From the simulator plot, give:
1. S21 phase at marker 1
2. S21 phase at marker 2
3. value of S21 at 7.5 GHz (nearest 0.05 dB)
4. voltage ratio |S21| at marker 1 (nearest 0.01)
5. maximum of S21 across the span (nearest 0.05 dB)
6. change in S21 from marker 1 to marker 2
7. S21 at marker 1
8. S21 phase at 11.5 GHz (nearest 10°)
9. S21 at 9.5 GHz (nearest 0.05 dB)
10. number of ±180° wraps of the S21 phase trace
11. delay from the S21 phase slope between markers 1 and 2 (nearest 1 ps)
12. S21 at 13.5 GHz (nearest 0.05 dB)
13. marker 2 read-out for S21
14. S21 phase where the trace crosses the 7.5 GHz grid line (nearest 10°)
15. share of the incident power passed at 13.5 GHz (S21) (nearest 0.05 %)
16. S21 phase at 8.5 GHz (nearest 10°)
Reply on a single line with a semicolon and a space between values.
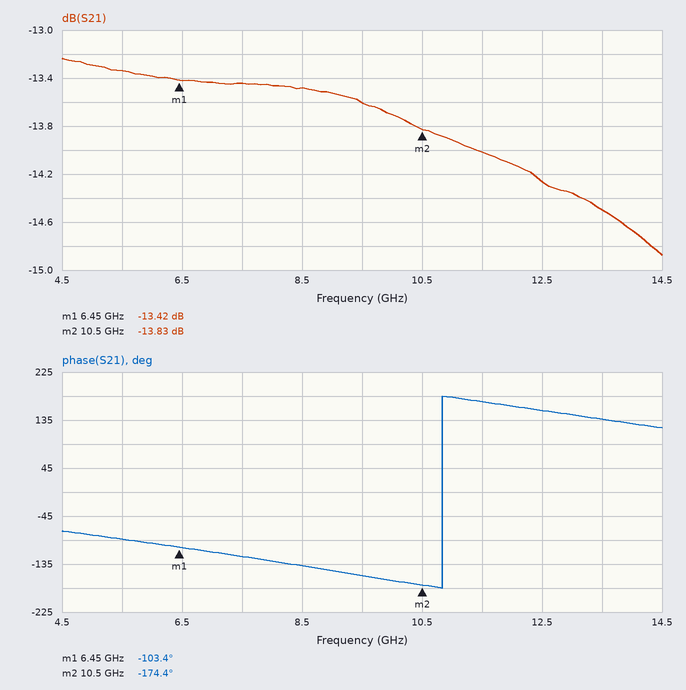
-103.4°; -174.4°; -13.45 dB; 0.21; -13.25 dB; -0.41 dB; -13.42 dB; 170°; -13.60 dB; 1; 49 ps; -14.50 dB; -13.83 dB; -120°; 3.55 %; -140°
